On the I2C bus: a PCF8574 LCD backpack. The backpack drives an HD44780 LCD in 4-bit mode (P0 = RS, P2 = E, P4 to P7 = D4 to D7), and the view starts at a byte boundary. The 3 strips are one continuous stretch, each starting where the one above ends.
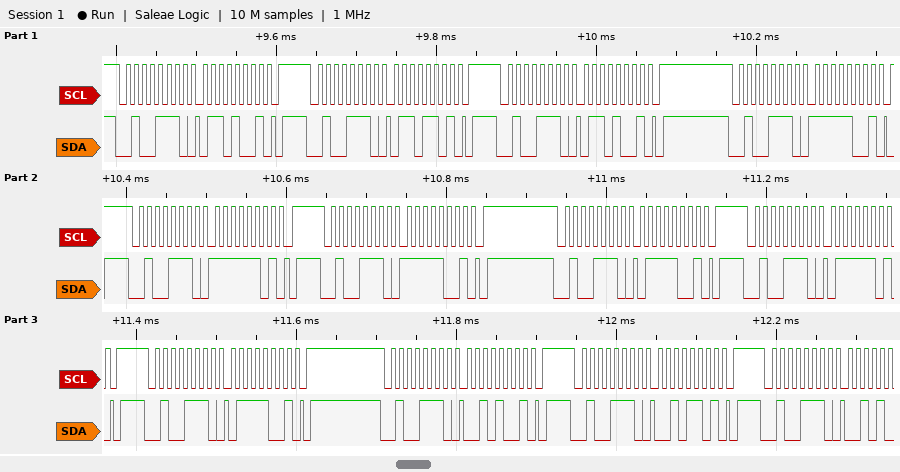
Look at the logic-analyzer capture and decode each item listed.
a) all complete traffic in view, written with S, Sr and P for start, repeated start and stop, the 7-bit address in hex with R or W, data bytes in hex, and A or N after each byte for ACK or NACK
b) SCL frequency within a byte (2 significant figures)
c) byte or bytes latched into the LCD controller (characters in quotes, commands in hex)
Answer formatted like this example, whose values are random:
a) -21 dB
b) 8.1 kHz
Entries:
a) S 27W A 69 A P S 27W A 6D A P S 27W A 69 A P S 27W A F9 A P S 27W A FD A P S 27W A F9 A P S 27W A 79 A P S 27W A 7D A P S 27W A 79 A P S 27W A 29 A P S 27W A 2D A P S 27W A
b) 100 kHz
c) 'o'
